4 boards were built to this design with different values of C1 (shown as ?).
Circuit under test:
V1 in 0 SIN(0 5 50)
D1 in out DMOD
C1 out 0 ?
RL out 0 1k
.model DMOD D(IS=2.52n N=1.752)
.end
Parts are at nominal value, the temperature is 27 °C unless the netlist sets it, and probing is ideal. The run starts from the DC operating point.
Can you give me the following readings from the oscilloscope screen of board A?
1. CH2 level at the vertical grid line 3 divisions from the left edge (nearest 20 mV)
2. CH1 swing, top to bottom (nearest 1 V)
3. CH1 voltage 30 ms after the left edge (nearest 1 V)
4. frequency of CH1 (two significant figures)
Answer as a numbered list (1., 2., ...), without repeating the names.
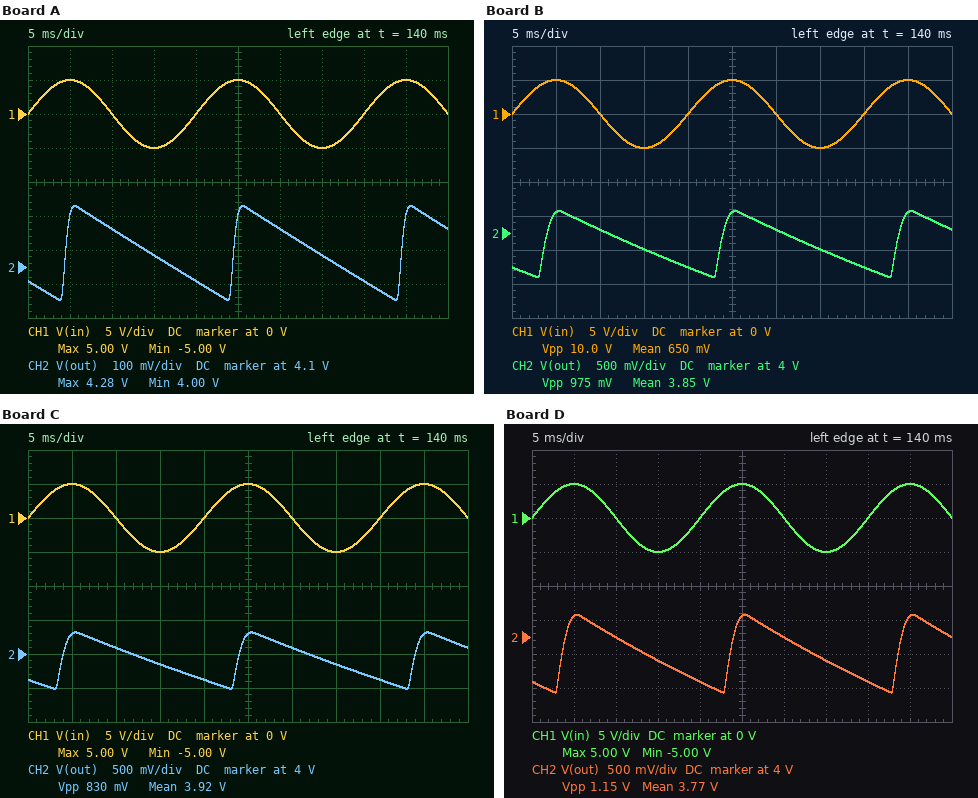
1. 4.14 V
2. 10 V
3. 0 V
4. 50 Hz
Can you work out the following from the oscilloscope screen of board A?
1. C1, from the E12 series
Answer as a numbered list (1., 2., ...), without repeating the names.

1. 270 µF
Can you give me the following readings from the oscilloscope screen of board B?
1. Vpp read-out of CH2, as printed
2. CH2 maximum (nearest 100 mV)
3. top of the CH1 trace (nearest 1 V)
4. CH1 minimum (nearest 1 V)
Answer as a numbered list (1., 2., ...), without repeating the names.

1. 975 mV
2. 4.3 V
3. 5 V
4. -5 V
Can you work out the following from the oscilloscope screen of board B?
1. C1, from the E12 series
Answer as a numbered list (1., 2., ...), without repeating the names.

1. 68 µF
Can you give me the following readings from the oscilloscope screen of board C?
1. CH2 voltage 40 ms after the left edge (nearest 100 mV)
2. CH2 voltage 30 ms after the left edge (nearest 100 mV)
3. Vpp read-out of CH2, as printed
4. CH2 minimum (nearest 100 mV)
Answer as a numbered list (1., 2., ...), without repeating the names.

1. 3.6 V
2. 4.1 V
3. 830 mV
4. 3.5 V
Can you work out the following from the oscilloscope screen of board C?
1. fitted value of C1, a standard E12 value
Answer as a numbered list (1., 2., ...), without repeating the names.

1. 82 µF
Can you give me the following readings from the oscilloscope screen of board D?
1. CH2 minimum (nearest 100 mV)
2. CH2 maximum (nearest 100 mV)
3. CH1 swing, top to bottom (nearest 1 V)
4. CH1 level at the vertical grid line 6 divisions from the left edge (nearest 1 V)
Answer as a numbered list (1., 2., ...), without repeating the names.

1. 3.2 V
2. 4.3 V
3. 10 V
4. 0 V
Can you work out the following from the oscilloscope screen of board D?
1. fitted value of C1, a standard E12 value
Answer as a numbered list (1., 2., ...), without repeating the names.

1. 56 µF
